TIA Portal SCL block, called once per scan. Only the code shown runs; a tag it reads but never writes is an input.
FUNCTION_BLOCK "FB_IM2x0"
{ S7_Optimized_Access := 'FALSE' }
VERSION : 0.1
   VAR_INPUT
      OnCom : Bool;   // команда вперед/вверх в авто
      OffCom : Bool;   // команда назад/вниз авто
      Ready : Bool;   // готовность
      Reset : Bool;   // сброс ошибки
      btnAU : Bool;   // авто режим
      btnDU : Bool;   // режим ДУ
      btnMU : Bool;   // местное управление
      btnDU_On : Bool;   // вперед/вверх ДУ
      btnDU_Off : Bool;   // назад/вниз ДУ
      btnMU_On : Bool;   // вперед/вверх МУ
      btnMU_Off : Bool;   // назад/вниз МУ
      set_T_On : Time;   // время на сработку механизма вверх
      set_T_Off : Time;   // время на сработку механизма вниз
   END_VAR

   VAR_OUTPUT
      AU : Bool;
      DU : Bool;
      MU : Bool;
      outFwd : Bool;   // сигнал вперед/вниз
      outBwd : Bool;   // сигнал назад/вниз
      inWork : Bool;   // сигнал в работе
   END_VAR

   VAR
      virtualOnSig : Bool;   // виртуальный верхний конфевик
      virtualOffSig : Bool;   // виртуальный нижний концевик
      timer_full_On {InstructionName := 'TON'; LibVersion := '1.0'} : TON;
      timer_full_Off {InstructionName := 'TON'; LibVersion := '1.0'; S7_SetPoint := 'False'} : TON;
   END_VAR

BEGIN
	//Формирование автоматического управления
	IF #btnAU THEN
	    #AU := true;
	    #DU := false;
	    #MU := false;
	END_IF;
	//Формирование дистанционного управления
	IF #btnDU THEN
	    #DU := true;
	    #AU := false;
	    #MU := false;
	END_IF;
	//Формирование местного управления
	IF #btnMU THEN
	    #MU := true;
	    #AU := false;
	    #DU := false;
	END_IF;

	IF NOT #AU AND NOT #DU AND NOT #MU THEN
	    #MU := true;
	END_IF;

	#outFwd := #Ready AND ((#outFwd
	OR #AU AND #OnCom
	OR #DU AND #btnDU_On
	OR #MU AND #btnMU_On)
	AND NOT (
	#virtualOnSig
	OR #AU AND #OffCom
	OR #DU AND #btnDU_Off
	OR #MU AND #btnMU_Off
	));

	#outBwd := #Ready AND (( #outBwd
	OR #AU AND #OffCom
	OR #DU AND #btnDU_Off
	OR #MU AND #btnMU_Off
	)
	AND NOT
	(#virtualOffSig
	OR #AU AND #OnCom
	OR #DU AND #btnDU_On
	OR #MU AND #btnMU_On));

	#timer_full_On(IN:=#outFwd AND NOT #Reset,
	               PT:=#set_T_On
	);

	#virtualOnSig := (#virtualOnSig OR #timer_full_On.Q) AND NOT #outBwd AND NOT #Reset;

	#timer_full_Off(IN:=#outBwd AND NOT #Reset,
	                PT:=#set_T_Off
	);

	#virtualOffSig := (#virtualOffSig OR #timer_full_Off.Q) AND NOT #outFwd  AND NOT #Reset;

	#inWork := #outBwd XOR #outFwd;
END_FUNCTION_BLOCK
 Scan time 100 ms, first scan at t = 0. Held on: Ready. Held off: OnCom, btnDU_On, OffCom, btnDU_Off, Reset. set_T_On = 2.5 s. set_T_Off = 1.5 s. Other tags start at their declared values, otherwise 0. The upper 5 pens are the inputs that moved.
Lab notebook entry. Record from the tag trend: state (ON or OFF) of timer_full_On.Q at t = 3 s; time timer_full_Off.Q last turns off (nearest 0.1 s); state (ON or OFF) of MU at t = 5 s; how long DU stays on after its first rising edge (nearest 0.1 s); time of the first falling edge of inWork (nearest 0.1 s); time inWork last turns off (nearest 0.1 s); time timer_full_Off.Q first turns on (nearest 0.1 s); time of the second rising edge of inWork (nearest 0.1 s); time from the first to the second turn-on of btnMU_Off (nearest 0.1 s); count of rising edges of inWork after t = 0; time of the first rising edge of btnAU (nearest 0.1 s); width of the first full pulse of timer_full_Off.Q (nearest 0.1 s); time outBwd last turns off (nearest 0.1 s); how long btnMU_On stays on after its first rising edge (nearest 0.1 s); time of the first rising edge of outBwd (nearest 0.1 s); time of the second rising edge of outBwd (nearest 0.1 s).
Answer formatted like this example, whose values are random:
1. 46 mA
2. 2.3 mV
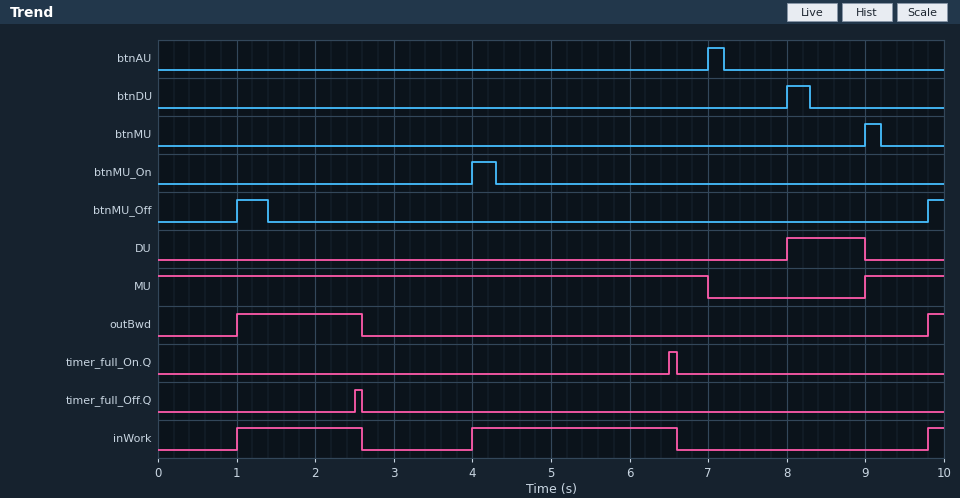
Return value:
1. OFF
2. 2.6 s
3. ON
4. 1.0 s
5. 2.6 s
6. 6.6 s
7. 2.5 s
8. 4.0 s
9. 8.8 s
10. 3
11. 7.0 s
12. 0.1 s
13. 2.6 s
14. 0.3 s
15. 1.0 s
16. 9.8 s
